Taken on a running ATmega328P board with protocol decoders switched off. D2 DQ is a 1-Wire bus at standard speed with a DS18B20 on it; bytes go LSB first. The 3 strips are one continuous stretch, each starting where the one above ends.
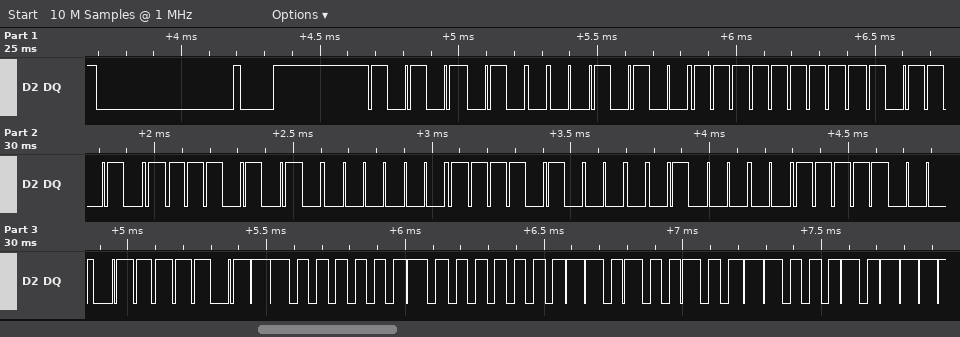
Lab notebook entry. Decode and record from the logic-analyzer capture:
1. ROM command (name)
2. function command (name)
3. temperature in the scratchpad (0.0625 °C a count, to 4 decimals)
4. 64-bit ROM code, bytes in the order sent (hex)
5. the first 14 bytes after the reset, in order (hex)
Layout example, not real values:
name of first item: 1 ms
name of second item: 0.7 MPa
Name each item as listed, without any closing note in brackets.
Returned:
ROM command: Match ROM
function command: Read Scratchpad
temperature in the scratchpad: 16.1875 °C
64-bit ROM code, bytes in the order sent: 28 FF 5B AF 80 17 04 1F
the first 14 bytes after the reset, in order: 55 28 FF 5B AF 80 17 04 1F BE 03 01 4B 46
